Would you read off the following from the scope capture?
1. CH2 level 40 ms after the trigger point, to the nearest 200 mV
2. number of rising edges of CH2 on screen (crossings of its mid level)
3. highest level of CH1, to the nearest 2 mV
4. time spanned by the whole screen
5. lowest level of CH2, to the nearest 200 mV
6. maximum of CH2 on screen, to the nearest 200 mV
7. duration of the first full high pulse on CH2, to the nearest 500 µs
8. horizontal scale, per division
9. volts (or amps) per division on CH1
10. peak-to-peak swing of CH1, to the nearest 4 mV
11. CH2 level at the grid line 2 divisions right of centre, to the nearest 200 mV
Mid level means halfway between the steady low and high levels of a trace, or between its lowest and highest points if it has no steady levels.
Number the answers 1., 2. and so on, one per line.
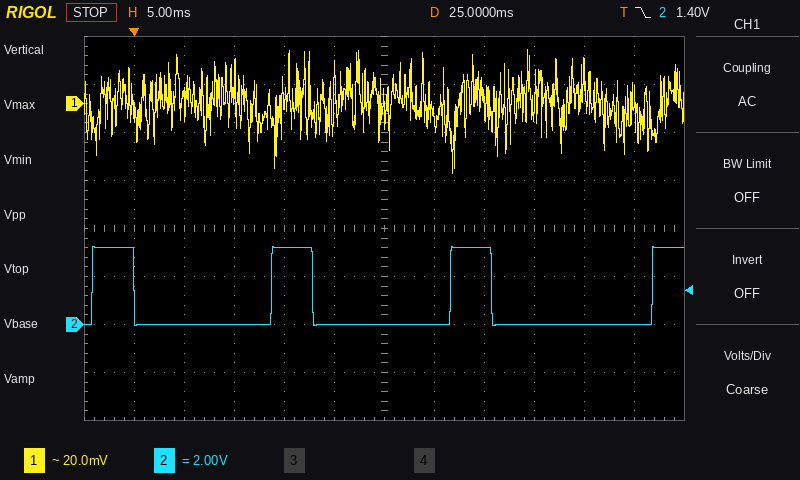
1. 0.0 V
2. 4
3. 22 mV
4. 60 ms
5. 0.0 V
6. 3.2 V
7. 4.0 ms
8. 5 ms
9. 20 mV
10. 52 mV
11. 3.2 V
